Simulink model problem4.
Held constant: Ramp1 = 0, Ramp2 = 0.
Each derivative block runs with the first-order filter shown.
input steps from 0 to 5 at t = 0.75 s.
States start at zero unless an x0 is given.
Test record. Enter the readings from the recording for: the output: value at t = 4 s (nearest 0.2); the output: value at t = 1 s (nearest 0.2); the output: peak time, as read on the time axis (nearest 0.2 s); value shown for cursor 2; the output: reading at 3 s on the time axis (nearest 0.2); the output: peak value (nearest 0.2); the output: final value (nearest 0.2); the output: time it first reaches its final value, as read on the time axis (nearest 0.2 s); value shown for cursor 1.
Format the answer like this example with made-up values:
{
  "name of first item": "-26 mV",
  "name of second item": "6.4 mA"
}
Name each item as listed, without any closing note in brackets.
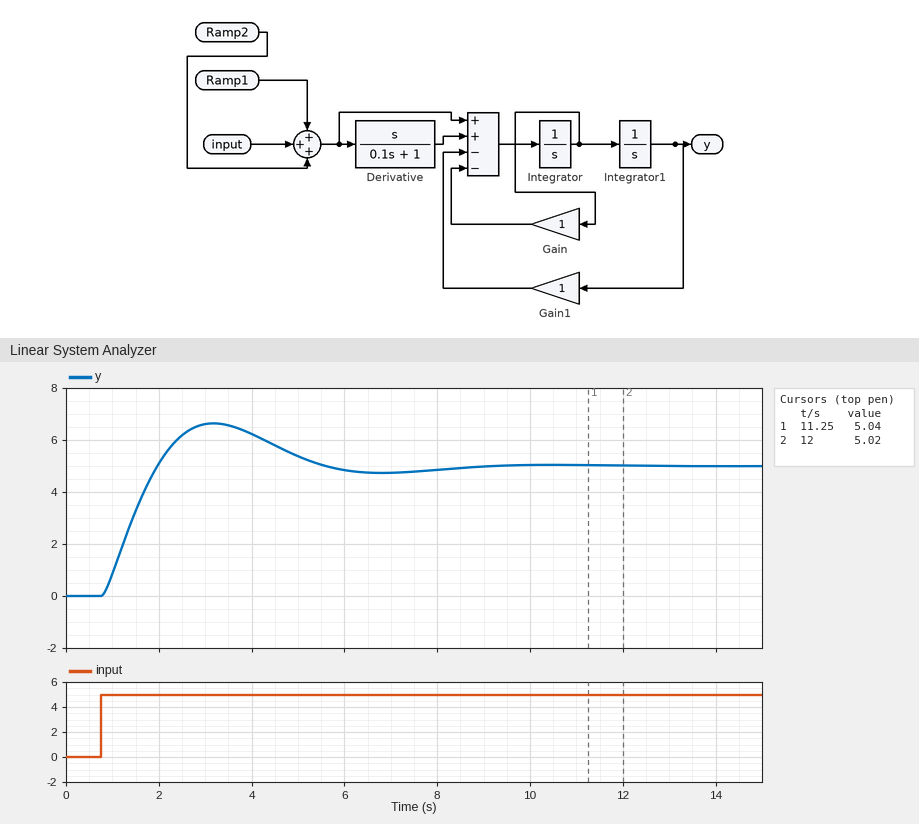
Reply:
{
  "the output: value at t = 4 s": "6.2",
  "the output: value at t = 1 s": "0.8",
  "the output: peak time, as read on the time axis": "3.2 s",
  "value shown for cursor 2": "5.02",
  "the output: reading at 3 s on the time axis": "6.6",
  "the output: peak value": "6.6",
  "the output: final value": "5.0",
  "the output: time it first reaches its final value, as read on the time axis": "2.0 s",
  "value shown for cursor 1": "5.04"
}
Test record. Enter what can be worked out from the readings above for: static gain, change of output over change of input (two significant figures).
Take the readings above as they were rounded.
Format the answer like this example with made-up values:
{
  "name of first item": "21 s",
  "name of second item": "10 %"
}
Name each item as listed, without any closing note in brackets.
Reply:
{
  "static gain, change of output over change of input": "1.0"
}
